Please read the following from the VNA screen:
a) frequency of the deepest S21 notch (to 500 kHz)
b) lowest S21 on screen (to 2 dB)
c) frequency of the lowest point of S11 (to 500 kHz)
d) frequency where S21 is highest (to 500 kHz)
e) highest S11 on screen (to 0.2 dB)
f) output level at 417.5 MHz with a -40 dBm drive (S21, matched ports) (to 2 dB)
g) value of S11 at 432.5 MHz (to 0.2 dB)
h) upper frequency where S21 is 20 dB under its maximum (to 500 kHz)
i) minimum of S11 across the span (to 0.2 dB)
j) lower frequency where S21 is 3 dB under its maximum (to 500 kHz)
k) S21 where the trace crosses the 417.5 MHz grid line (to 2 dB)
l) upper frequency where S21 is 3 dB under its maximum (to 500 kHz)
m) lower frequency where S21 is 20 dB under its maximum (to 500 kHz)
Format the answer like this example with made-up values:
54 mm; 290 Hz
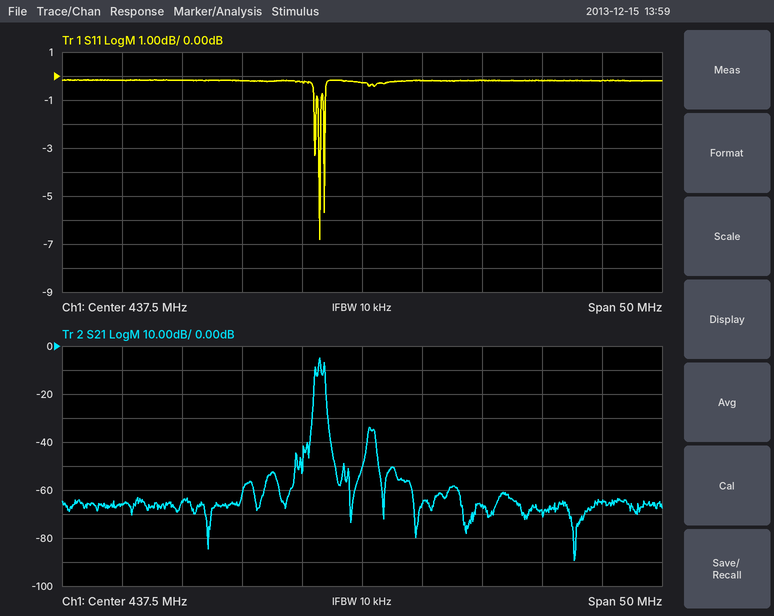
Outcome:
455.0 MHz; -90 dB; 434.0 MHz; 434.0 MHz; -0.2 dB; -106 dBm; -0.2 dB; 434.5 MHz; -6.8 dB; 434.0 MHz; -66 dB; 434.0 MHz; 433.5 MHz
